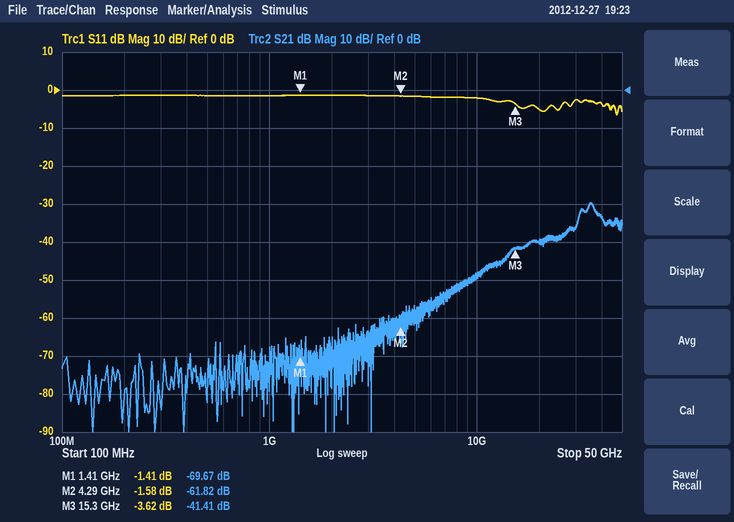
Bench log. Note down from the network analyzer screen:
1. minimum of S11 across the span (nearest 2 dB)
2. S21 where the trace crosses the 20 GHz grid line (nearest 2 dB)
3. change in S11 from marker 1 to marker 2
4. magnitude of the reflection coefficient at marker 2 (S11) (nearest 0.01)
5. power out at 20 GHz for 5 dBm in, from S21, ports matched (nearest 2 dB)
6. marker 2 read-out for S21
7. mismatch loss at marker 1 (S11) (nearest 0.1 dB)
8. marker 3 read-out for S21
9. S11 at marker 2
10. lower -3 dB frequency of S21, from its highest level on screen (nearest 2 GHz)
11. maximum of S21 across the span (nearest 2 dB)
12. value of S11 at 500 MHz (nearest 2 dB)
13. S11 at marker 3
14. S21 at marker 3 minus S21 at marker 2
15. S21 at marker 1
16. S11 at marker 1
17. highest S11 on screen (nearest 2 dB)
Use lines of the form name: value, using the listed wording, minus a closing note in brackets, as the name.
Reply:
minimum of S11 across the span: -6 dB
S21 where the trace crosses the 20 GHz grid line: -40 dB
change in S11 from marker 1 to marker 2: -0.17 dB
magnitude of the reflection coefficient at marker 2 (S11): 0.83
power out at 20 GHz for 5 dBm in, from S21, ports matched: -36 dBm
marker 2 read-out for S21: -61.82 dB
mismatch loss at marker 1 (S11): 5.6 dB
marker 3 read-out for S21: -41.41 dB
S11 at marker 2: -1.58 dB
lower -3 dB frequency of S21, from its highest level on screen: 32 GHz
maximum of S21 across the span: -30 dB
value of S11 at 500 MHz: -2 dB
S11 at marker 3: -3.62 dB
S21 at marker 3 minus S21 at marker 2: 20.41 dB
S21 at marker 1: -69.67 dB
S11 at marker 1: -1.41 dB
highest S11 on screen: -2 dB
